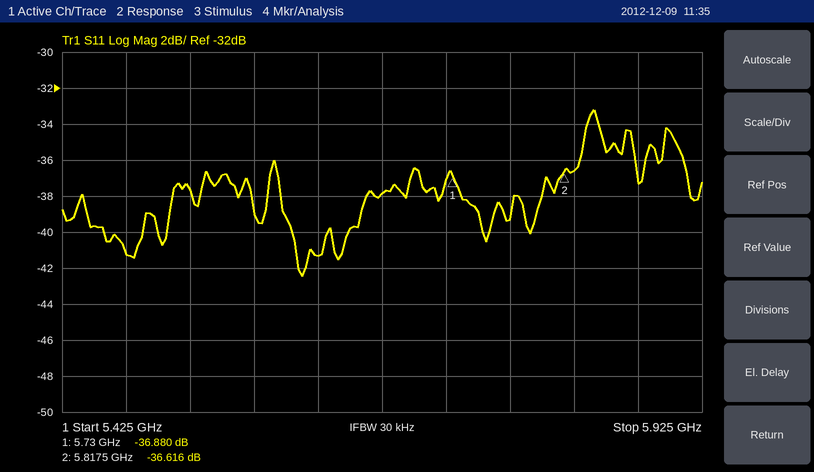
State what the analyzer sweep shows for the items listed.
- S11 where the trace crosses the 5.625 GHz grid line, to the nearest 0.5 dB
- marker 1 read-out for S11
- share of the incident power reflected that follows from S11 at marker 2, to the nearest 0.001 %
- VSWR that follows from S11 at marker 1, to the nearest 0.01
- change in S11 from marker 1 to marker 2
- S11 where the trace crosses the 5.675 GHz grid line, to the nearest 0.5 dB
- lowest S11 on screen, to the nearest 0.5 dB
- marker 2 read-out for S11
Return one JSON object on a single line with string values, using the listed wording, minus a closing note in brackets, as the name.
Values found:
{"S11 where the trace crosses the 5.625 GHz grid line, to the nearest 0.5 dB": "-41.5 dB", "marker 1 read-out for S11": "-36.880 dB", "share of the incident power reflected that follows from S11 at marker 2, to the nearest 0.001 %": "0.022 %", "VSWR that follows from S11 at marker 1, to the nearest 0.01": "1.03", "change in S11 from marker 1 to marker 2": "0.264 dB", "S11 where the trace crosses the 5.675 GHz grid line, to the nearest 0.5 dB": "-38.0 dB", "lowest S11 on screen, to the nearest 0.5 dB": "-42.5 dB", "marker 2 read-out for S11": "-36.616 dB"}
